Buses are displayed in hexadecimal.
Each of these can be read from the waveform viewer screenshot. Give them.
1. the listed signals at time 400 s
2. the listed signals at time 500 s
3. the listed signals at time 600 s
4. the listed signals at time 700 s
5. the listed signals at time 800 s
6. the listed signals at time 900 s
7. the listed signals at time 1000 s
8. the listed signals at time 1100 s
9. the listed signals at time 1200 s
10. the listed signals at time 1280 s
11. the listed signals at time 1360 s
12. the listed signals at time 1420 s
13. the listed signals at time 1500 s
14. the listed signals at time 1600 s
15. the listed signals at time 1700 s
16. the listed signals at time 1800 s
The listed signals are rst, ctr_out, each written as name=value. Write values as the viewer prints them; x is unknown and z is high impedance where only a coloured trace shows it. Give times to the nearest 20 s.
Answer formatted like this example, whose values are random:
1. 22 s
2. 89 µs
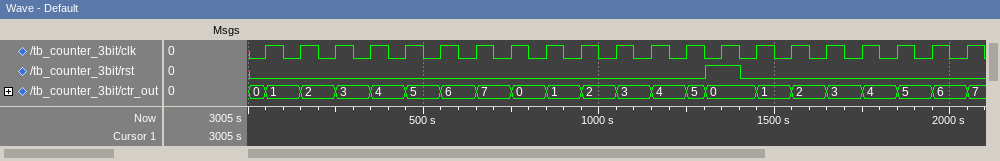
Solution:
1. rst=0, ctr_out=4
2. rst=0, ctr_out=5
3. rst=0, ctr_out=6
4. rst=0, ctr_out=7
5. rst=0, ctr_out=0
6. rst=0, ctr_out=1
7. rst=0, ctr_out=2
8. rst=0, ctr_out=3
9. rst=0, ctr_out=4
10. rst=0, ctr_out=5
11. rst=1, ctr_out=0
12. rst=0, ctr_out=0
13. rst=0, ctr_out=1
14. rst=0, ctr_out=2
15. rst=0, ctr_out=3
16. rst=0, ctr_out=4
